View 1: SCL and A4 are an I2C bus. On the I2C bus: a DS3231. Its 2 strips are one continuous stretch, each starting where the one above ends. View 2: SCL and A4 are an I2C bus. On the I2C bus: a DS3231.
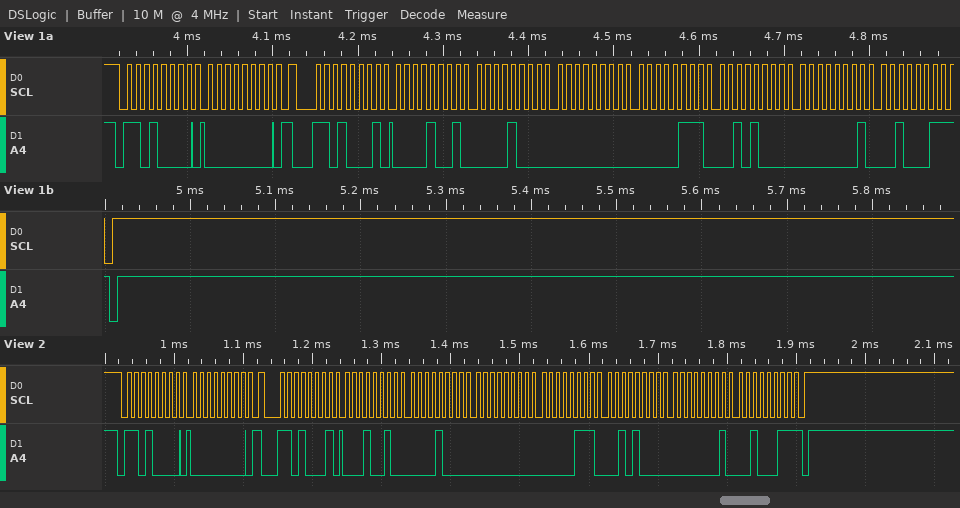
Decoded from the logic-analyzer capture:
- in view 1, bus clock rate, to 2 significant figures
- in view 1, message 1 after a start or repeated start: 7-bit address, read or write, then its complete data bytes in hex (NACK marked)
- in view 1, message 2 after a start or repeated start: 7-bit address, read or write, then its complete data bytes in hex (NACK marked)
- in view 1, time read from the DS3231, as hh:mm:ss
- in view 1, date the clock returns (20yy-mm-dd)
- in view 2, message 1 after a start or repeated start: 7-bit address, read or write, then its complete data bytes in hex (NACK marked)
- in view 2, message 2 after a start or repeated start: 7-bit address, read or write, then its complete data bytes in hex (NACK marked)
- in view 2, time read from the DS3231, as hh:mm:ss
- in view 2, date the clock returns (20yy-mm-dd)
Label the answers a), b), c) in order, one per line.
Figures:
a) 100 kHz
b) 0x68 write: 00
c) 0x68 read: 09 08 00 07 28 01 23 NACK
d) 00:08:09
e) 2023-01-28
f) 0x68 write: 00
g) 0x68 read: 12 08 00 07 28 01 23 NACK
h) 00:08:12
i) 2023-01-28
